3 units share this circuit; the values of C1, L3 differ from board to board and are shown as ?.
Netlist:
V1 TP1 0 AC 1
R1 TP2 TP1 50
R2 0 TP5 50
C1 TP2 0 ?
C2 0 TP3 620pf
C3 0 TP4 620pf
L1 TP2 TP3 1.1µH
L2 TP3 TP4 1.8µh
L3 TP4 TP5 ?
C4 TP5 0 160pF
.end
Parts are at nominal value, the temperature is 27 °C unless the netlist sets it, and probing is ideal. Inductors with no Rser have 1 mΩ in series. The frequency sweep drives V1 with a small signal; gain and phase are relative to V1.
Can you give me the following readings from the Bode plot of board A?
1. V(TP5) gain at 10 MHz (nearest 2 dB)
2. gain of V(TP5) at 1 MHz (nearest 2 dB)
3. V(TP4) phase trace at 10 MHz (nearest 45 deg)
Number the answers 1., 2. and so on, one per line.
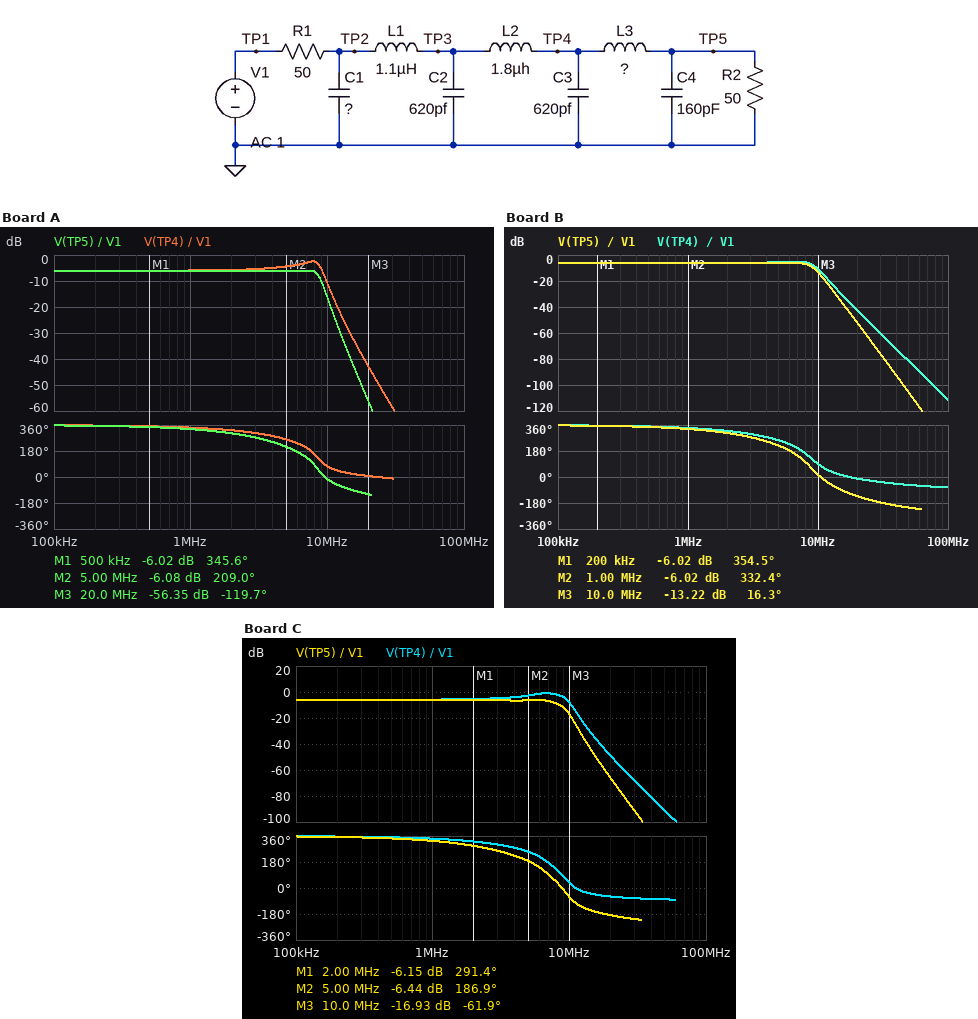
1. -16 dB
2. -6 dB
3. 90 deg
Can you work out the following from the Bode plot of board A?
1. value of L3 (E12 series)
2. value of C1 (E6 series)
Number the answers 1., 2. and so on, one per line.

1. 1.5 µH
2. 47 pF
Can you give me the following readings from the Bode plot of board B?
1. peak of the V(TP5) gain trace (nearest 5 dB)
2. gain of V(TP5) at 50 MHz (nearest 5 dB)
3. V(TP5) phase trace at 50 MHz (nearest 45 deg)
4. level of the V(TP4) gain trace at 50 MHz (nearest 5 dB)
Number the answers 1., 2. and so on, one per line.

1. -5 dB
2. -105 dB
3. -225 deg
4. -80 dB
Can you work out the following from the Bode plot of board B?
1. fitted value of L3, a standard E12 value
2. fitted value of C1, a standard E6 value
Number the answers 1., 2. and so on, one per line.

1. 1 µH
2. 100 pF
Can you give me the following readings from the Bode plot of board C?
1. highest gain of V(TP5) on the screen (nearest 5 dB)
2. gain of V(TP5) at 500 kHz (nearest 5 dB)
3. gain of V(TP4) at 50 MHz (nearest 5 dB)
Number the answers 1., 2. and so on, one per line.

1. -5 dB
2. -5 dB
3. -90 dB
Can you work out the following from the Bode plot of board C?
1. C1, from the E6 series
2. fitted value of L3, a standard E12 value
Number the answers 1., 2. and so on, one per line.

1. 330 pF
2. 2.2 µH
